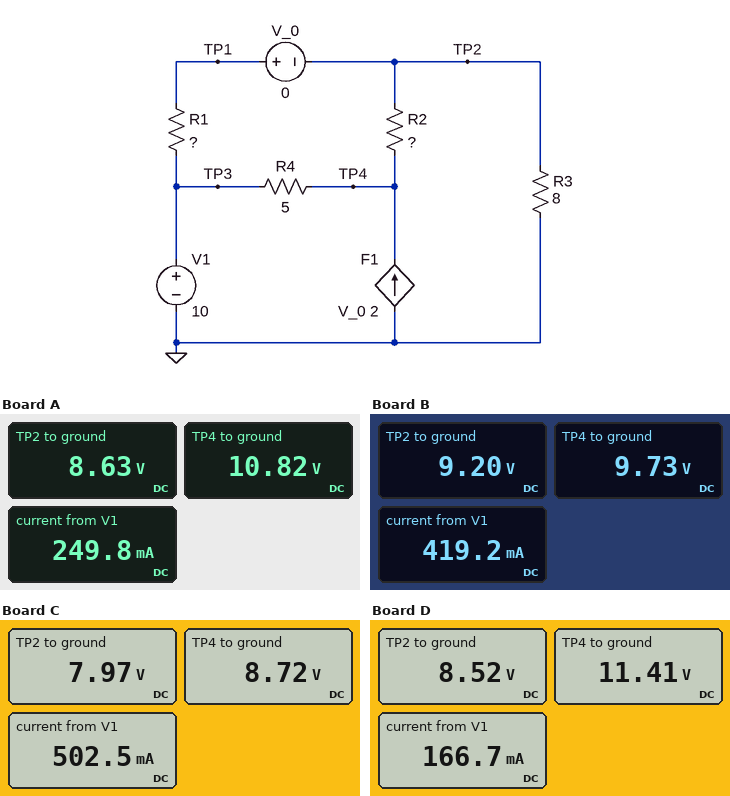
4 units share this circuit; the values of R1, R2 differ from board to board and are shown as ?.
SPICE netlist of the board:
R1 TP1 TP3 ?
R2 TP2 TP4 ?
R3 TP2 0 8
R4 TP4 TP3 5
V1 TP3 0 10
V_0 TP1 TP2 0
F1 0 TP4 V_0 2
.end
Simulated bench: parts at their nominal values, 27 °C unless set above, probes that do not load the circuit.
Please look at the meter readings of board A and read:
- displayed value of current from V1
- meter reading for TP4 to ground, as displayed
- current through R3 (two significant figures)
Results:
249.8 mA
10.82 V
1.1 A
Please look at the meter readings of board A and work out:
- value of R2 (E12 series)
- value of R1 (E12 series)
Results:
3.3 Ω
3.3 Ω
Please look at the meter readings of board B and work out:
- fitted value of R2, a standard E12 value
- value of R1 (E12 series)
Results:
0.68 Ω
2.2 Ω
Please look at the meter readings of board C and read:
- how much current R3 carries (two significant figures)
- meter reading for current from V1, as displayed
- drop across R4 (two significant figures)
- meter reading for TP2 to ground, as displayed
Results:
1.0 A
502.5 mA
1.3 V
7.97 V
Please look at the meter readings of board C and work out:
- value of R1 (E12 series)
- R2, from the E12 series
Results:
8.2 Ω
1 Ω
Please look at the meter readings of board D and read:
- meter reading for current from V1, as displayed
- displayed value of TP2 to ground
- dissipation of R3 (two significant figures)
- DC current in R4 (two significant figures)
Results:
166.7 mA
8.52 V
9.1 W
280 mA
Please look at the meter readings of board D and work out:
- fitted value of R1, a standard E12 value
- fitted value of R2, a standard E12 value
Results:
3.3 Ω
4.7 Ω
